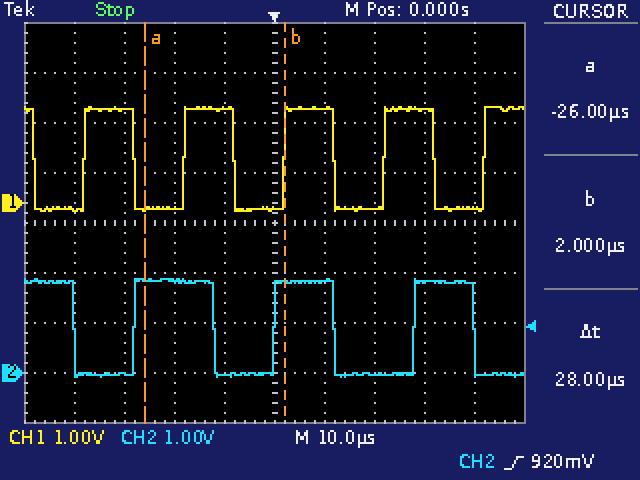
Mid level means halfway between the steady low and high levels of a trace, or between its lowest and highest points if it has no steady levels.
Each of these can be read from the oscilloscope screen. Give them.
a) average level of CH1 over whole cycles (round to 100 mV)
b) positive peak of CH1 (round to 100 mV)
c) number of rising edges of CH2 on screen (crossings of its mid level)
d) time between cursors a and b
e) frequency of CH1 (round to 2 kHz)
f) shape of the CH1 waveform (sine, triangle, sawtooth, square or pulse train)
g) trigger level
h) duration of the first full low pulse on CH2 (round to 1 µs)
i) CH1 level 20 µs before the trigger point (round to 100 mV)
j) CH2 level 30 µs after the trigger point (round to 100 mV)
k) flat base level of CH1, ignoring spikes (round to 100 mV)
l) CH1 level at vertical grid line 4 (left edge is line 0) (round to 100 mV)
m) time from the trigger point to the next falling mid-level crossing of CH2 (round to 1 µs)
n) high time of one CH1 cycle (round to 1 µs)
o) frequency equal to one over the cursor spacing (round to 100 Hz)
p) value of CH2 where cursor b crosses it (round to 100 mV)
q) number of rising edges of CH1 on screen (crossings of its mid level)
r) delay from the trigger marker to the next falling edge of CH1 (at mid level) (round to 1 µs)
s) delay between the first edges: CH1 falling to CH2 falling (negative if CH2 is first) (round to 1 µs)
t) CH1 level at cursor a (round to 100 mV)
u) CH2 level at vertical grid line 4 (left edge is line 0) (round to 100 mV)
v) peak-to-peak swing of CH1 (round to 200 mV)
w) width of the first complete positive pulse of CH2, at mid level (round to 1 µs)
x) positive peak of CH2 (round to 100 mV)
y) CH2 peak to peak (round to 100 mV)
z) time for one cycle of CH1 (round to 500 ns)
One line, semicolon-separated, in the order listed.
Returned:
900 mV; 1.9 V; 3; 28 µs; 50 kHz; square; 920 mV; 12 µs; -100 mV; 1.8 V; -100 mV; 1.9 V; 12 µs; 10 µs; 35.7 kHz; 1.8 V; 5; 12 µs; +8 µs; -100 mV; 0.0 V; 2.0 V; 16 µs; 1.9 V; 2.0 V; 20.0 µs
